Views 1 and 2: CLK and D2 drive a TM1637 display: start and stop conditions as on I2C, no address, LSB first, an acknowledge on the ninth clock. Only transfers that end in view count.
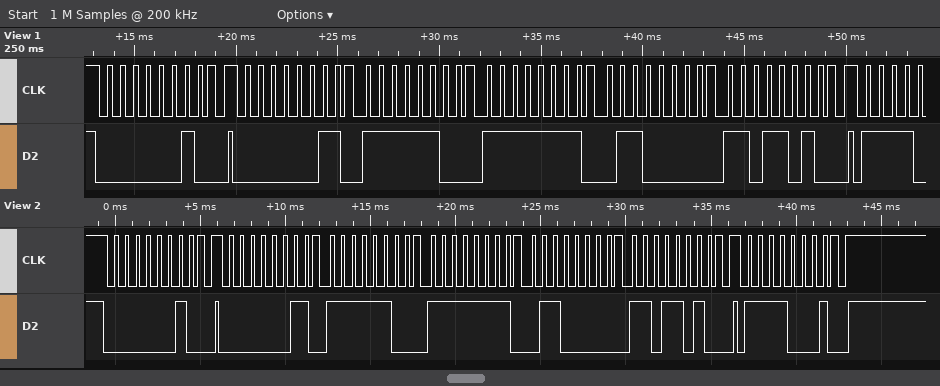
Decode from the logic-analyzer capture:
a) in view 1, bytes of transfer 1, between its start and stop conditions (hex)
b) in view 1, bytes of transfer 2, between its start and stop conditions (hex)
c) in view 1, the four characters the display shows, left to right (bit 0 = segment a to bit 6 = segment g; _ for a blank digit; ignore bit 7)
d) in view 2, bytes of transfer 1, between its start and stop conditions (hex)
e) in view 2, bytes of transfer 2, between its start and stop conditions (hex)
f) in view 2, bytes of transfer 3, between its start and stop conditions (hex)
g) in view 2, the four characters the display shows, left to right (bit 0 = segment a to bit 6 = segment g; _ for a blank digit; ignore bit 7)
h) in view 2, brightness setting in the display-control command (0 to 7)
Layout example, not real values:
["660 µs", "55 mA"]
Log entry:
["40", "C0 3F FF 06 5B", "0812", "40", "C0 3F FF 06 5B", "8F", "0812", "7"]
